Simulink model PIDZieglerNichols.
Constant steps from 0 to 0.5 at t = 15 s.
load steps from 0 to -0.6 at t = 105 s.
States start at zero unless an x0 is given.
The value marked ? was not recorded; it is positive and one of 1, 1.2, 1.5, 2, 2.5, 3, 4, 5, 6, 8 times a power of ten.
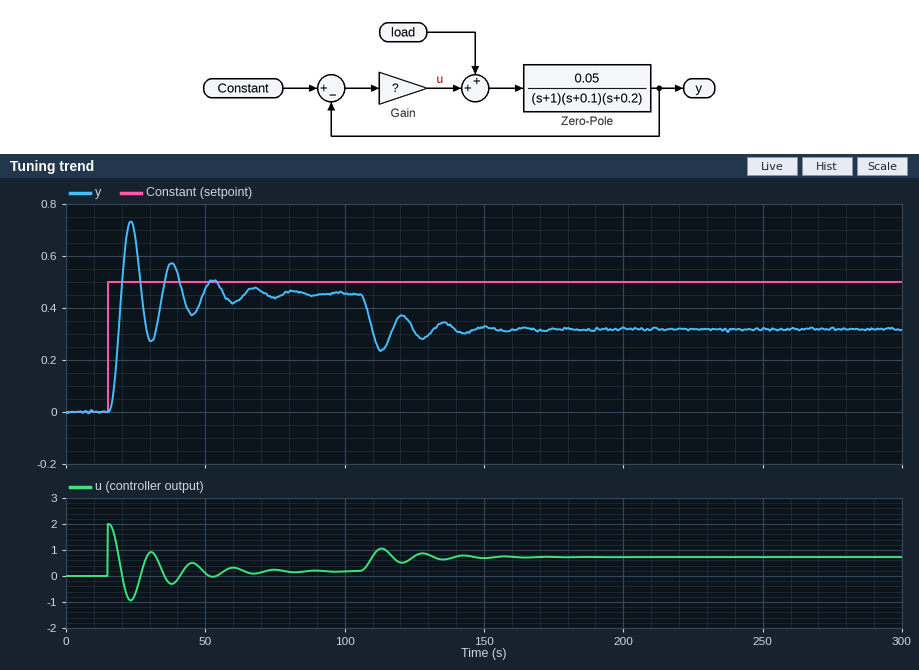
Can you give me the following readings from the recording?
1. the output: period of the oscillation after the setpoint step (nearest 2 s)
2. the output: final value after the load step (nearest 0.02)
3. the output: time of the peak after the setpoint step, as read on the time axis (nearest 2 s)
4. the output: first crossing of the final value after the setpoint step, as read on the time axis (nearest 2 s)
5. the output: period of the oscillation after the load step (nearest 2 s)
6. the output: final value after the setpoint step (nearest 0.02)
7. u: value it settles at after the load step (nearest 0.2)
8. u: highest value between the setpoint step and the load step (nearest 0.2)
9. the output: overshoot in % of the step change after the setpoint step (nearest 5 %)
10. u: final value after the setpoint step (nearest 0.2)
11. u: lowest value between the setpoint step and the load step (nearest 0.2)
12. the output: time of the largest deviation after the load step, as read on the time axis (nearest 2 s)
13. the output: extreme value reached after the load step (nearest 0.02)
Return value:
14 s
0.32
24 s
20 s
14 s
0.46
0.8
2.0
60 %
0.2
-1.0
114 s
0.24
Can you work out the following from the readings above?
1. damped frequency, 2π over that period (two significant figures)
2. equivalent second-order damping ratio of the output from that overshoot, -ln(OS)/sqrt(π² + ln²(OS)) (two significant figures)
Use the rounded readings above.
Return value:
0.45 rad/s
0.16
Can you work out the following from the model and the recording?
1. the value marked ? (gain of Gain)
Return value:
4
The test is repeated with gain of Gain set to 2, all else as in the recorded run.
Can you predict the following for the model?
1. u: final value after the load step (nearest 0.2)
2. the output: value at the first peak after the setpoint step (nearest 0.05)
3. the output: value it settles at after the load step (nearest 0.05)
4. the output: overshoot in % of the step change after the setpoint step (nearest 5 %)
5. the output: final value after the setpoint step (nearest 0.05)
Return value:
0.6
0.55
0.15
35 %
0.40
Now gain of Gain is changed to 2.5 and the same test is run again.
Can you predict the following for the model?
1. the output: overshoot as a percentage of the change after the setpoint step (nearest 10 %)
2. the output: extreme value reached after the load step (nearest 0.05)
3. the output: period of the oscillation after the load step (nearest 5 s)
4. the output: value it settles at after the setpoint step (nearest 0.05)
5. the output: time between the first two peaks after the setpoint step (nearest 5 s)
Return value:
40 %
0.15
20 s
0.45
20 s
